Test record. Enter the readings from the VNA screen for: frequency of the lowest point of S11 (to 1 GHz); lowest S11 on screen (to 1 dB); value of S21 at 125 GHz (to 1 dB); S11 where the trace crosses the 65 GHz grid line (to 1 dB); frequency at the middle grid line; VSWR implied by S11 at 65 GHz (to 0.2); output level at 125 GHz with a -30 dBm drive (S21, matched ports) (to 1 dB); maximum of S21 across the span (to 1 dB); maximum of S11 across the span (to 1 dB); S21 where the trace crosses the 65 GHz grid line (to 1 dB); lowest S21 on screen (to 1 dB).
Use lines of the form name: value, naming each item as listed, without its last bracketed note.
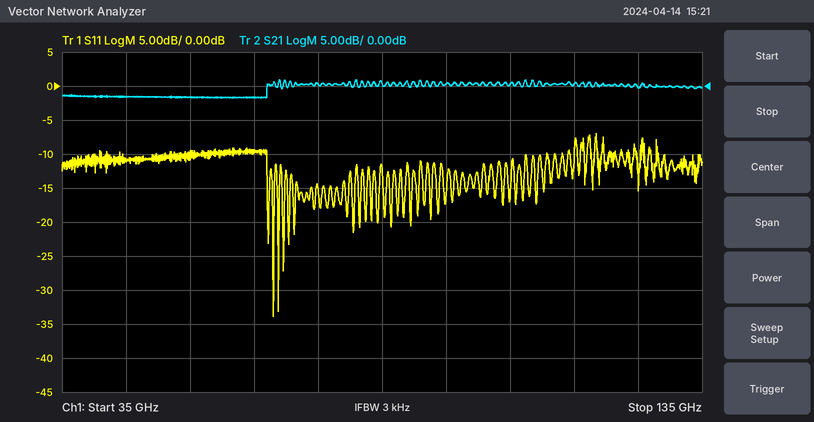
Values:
frequency of the lowest point of S11: 68 GHz
lowest S11 on screen: -34 dB
value of S21 at 125 GHz: 0 dB
S11 where the trace crosses the 65 GHz grid line: -10 dB
frequency at the middle grid line: 85 GHz
VSWR implied by S11 at 65 GHz: 2.0
output level at 125 GHz with a -30 dBm drive (S21, matched ports): -30 dBm
maximum of S21 across the span: 1 dB
maximum of S11 across the span: -7 dB
S21 where the trace crosses the 65 GHz grid line: -2 dB
lowest S21 on screen: -2 dB
